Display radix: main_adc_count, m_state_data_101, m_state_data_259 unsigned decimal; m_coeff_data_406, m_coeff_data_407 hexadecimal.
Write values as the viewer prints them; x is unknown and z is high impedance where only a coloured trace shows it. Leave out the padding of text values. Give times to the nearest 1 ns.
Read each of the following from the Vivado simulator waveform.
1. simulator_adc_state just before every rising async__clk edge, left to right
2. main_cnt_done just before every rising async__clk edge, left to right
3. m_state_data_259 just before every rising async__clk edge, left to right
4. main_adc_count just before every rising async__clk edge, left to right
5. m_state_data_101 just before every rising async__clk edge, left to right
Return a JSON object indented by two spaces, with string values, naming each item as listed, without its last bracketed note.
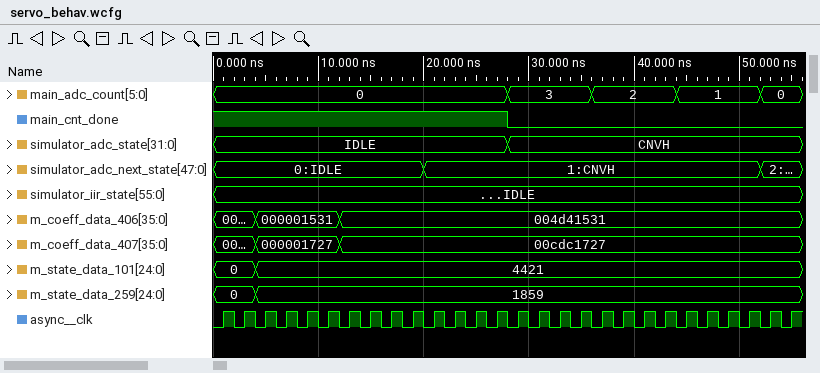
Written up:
{
  "simulator_adc_state just before every rising async__clk edge, left to right": "IDLE, IDLE, IDLE, IDLE, IDLE, IDLE, IDLE, IDLE, IDLE, IDLE, IDLE, IDLE, IDLE, IDLE, CNVH, CNVH, CNVH, CNVH, CNVH, CNVH, CNVH, CNVH, CNVH, CNVH, CNVH, CNVH, CNVH, CNVH",
  "main_cnt_done just before every rising async__clk edge, left to right": "1 1 1 1 1 1 1 1 1 1 1 1 1 1 0 0 0 0 0 0 0 0 0 0 0 0 0 0",
  "m_state_data_259 just before every rising async__clk edge, left to right": "0, 0, 1859, 1859, 1859, 1859, 1859, 1859, 1859, 1859, 1859, 1859, 1859, 1859, 1859, 1859, 1859, 1859, 1859, 1859, 1859, 1859, 1859, 1859, 1859, 1859, 1859, 1859",
  "main_adc_count just before every rising async__clk edge, left to right": "0, 0, 0, 0, 0, 0, 0, 0, 0, 0, 0, 0, 0, 0, 3, 3, 3, 3, 2, 2, 2, 2, 1, 1, 1, 1, 0, 0",
  "m_state_data_101 just before every rising async__clk edge, left to right": "0, 0, 4421, 4421, 4421, 4421, 4421, 4421, 4421, 4421, 4421, 4421, 4421, 4421, 4421, 4421, 4421, 4421, 4421, 4421, 4421, 4421, 4421, 4421, 4421, 4421, 4421, 4421"
}
